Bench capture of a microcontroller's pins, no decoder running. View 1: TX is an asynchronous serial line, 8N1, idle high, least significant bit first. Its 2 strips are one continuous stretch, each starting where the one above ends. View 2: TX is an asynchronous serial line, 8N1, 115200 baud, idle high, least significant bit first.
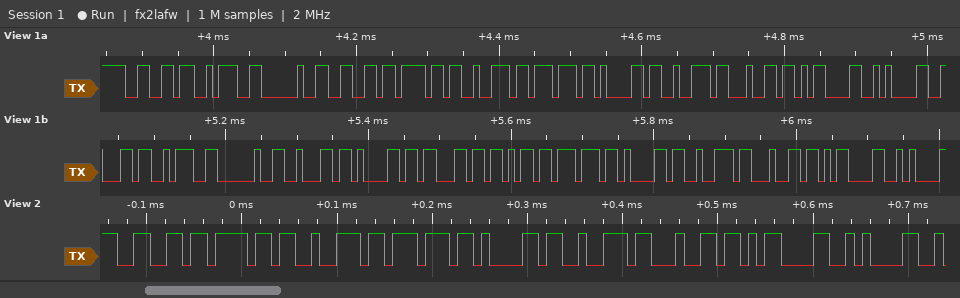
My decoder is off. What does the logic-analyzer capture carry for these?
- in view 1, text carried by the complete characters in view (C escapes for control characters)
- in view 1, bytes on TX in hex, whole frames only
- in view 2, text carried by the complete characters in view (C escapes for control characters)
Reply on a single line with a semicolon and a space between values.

"f: forward\r\nb: backward\r\n"; 0x66 0x3A 0x20 0x66 0x6F 0x72 0x77 0x61 0x72 0x64 0x0D 0x0A 0x62 0x3A 0x20 0x62 0x61 0x63 0x6B 0x77 0x61 0x72 0x64 0x0D 0x0A; "forward\r\n"
